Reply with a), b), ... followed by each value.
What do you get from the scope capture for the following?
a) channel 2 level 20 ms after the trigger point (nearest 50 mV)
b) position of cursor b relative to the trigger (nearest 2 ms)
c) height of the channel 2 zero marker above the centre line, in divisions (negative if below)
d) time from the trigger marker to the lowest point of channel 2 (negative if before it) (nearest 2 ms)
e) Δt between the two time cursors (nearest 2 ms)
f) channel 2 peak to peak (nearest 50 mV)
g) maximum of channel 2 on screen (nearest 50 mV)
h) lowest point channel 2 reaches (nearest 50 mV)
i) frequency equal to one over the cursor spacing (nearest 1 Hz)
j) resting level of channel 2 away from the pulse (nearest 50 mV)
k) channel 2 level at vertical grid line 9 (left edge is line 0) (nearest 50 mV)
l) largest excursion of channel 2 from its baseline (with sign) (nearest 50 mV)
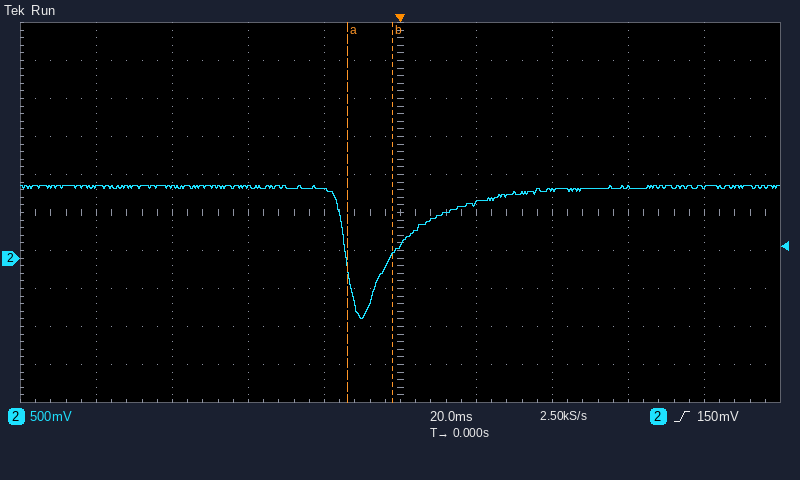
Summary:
a) 700 mV
b) -2 ms
c) -1.2 div
d) -10 ms
e) 12 ms
f) 1.75 V
g) 950 mV
h) -800 mV
i) 83 Hz
j) 950 mV
k) 950 mV
l) -1.75 V
